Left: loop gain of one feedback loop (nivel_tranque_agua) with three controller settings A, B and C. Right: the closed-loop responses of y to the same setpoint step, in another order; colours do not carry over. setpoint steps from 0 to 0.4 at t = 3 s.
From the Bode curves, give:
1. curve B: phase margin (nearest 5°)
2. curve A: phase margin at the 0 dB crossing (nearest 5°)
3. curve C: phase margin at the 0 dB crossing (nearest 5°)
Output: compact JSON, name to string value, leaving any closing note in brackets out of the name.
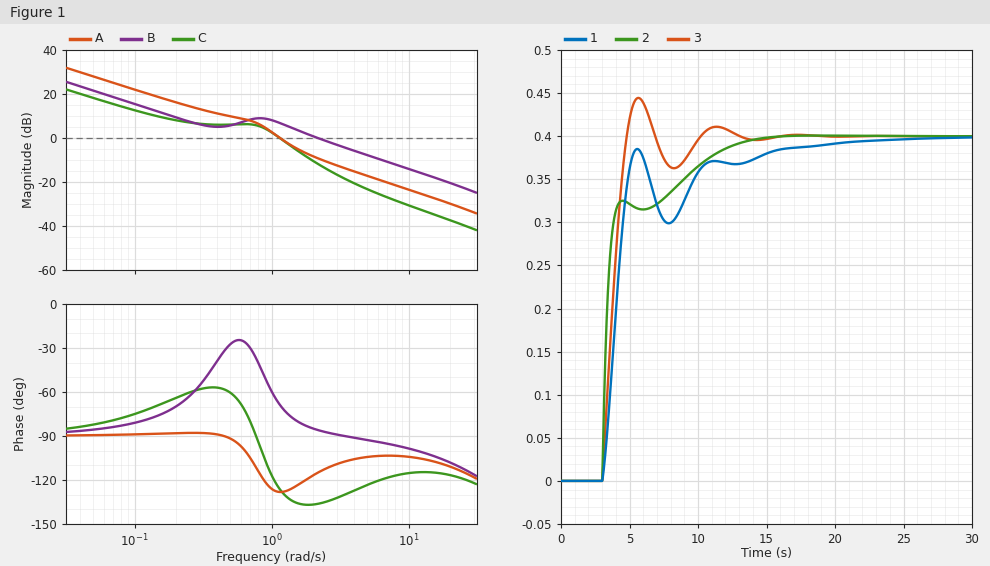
{"curve B: phase margin": "95°", "curve A: phase margin at the 0 dB crossing": "50°", "curve C: phase margin at the 0 dB crossing": "55°"}
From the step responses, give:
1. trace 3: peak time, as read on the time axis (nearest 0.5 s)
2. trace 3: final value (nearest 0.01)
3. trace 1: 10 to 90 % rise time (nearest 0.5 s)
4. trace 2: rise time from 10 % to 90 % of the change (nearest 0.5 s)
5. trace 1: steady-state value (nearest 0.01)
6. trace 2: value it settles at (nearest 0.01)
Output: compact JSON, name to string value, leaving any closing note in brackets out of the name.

{"trace 3: peak time, as read on the time axis": "5.5 s", "trace 3: final value": "0.40", "trace 1: 10 to 90 % rise time": "1.5 s", "trace 2: rise time from 10 % to 90 % of the change": "6.5 s", "trace 1: steady-state value": "0.40", "trace 2: value it settles at": "0.40"}
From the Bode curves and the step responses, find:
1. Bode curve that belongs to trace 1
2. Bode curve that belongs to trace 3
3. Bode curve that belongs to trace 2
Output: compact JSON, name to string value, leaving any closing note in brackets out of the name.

{"Bode curve that belongs to trace 1": "C", "Bode curve that belongs to trace 3": "A", "Bode curve that belongs to trace 2": "B"}
